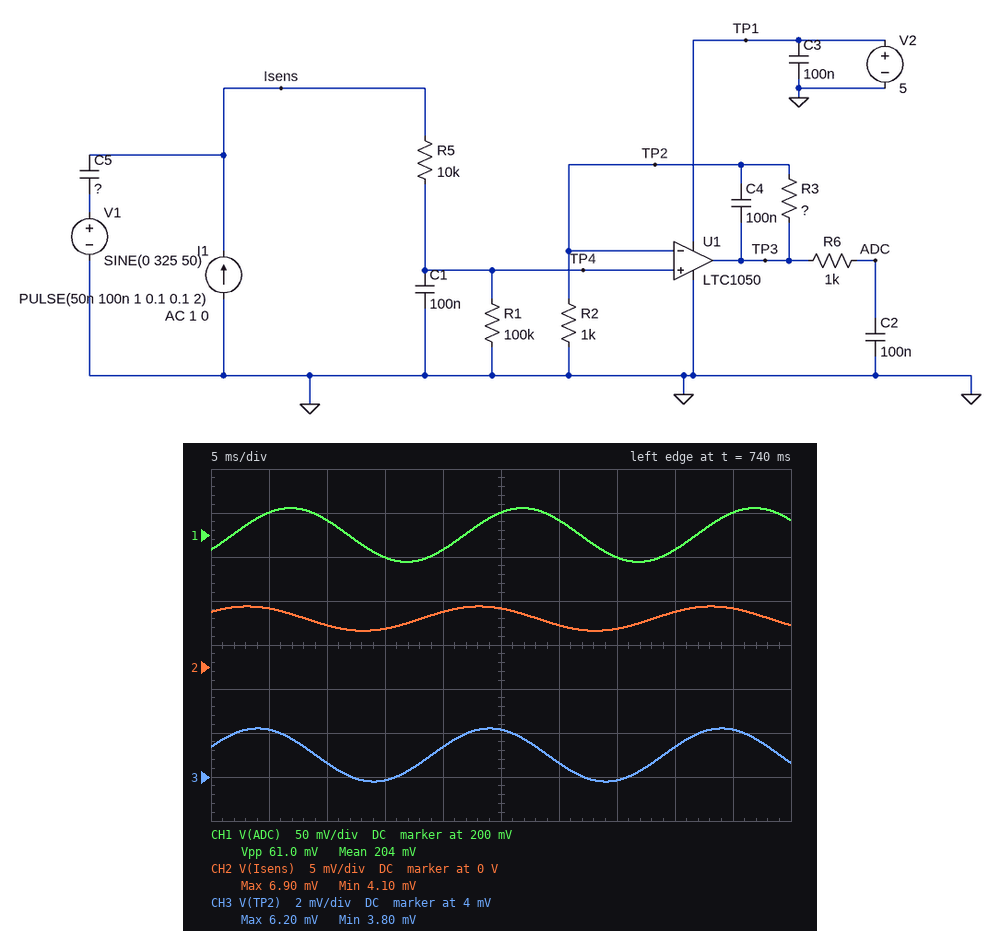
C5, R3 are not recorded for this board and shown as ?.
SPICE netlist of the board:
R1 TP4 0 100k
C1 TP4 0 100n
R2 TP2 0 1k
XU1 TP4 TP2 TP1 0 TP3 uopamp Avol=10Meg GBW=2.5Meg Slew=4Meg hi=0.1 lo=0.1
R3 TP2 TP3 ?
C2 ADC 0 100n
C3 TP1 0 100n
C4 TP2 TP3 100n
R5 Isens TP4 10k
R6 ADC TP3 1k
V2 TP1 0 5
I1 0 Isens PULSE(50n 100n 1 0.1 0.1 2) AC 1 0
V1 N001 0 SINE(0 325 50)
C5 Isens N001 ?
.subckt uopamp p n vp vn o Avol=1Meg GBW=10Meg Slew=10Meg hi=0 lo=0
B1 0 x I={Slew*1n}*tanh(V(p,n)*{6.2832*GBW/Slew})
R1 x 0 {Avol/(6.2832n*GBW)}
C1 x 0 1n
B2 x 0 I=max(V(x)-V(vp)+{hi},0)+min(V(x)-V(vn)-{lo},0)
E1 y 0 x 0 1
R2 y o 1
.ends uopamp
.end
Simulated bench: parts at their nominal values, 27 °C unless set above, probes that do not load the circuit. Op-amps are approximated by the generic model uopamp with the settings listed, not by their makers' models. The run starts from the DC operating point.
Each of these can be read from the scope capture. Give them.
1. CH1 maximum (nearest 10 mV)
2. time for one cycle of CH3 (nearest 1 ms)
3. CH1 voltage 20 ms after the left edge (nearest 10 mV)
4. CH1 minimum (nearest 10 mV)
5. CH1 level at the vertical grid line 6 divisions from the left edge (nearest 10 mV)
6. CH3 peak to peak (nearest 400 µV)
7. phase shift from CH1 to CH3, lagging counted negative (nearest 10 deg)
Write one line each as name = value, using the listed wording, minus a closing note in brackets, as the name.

CH1 maximum = 230 mV
time for one cycle of CH3 = 20 ms
CH1 voltage 20 ms after the left edge = 180 mV
CH1 minimum = 170 mV
CH1 level at the vertical grid line 6 divisions from the left edge = 220 mV
CH3 peak to peak = 2.4 mV
phase shift from CH1 to CH3, lagging counted negative = 50 deg
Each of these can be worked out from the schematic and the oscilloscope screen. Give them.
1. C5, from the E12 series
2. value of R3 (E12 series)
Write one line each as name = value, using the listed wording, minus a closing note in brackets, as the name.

C5, from the E12 series = 390 fF
value of R3 = 39 kΩ
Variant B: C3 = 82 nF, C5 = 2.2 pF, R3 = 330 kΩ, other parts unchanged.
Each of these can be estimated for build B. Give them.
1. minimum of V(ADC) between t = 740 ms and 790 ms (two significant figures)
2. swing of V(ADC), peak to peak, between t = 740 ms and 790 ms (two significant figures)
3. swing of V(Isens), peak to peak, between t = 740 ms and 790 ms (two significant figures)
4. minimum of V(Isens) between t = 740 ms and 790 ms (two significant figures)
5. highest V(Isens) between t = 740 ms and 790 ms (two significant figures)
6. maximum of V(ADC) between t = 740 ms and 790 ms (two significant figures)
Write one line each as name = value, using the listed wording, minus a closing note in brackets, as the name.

minimum of V(ADC) between t = 740 ms and 790 ms = 1.4 V
swing of V(ADC), peak to peak, between t = 740 ms and 790 ms = 430 mV
swing of V(Isens), peak to peak, between t = 740 ms and 790 ms = 16 mV
minimum of V(Isens) between t = 740 ms and 790 ms = -2.3 mV
highest V(Isens) between t = 740 ms and 790 ms = 13 mV
maximum of V(ADC) between t = 740 ms and 790 ms = 1.9 V
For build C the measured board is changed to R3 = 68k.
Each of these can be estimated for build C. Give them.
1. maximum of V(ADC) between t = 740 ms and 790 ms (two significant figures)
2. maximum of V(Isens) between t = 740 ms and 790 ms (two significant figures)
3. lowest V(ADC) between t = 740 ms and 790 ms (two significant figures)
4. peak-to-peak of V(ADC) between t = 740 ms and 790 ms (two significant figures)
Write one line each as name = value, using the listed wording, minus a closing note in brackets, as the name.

maximum of V(ADC) between t = 740 ms and 790 ms = 380 mV
maximum of V(Isens) between t = 740 ms and 790 ms = 6.9 mV
lowest V(ADC) between t = 740 ms and 790 ms = 310 mV
peak-to-peak of V(ADC) between t = 740 ms and 790 ms = 71 mV
